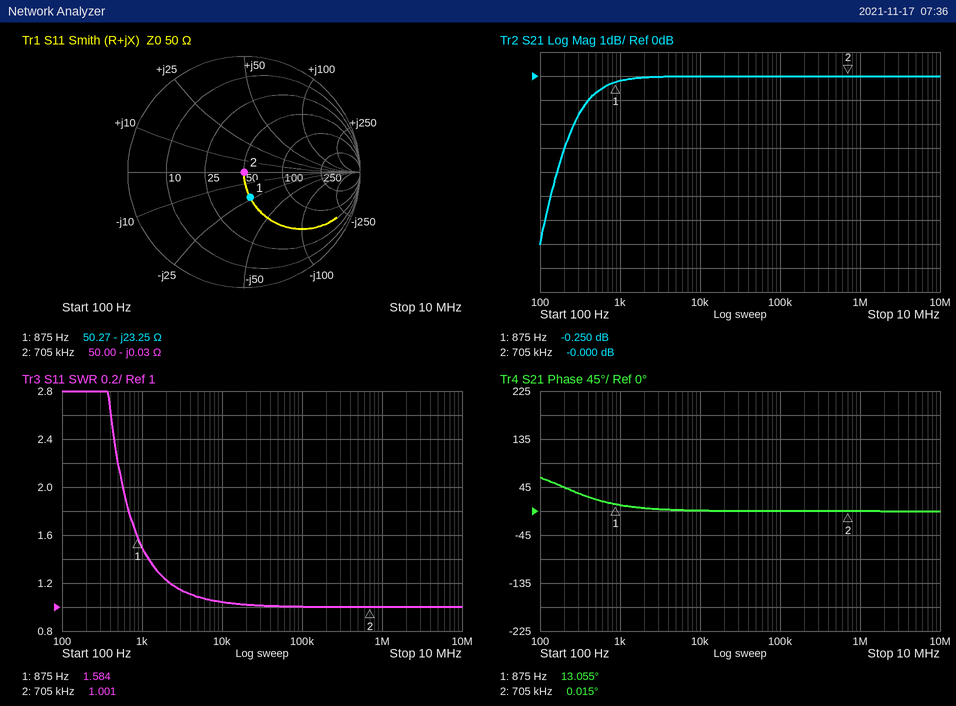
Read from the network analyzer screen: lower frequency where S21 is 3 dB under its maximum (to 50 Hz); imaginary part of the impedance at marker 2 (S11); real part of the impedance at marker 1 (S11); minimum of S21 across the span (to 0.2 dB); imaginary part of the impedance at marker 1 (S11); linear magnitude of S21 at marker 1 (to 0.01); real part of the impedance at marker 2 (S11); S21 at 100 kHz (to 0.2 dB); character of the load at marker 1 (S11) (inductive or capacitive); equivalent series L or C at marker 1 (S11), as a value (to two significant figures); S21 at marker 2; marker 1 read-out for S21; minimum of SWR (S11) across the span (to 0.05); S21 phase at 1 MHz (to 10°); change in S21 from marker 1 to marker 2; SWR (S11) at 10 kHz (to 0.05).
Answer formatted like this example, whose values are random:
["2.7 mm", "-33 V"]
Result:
["200 Hz", "-0.03 Ω", "50.27 Ω", "-7.0 dB", "-23.25 Ω", "0.97", "50.00 Ω", "0.0 dB", "capacitive", "7.8 µF", "-0.000 dB", "-0.250 dB", "1.00", "0°", "0.250 dB", "1.05"]
